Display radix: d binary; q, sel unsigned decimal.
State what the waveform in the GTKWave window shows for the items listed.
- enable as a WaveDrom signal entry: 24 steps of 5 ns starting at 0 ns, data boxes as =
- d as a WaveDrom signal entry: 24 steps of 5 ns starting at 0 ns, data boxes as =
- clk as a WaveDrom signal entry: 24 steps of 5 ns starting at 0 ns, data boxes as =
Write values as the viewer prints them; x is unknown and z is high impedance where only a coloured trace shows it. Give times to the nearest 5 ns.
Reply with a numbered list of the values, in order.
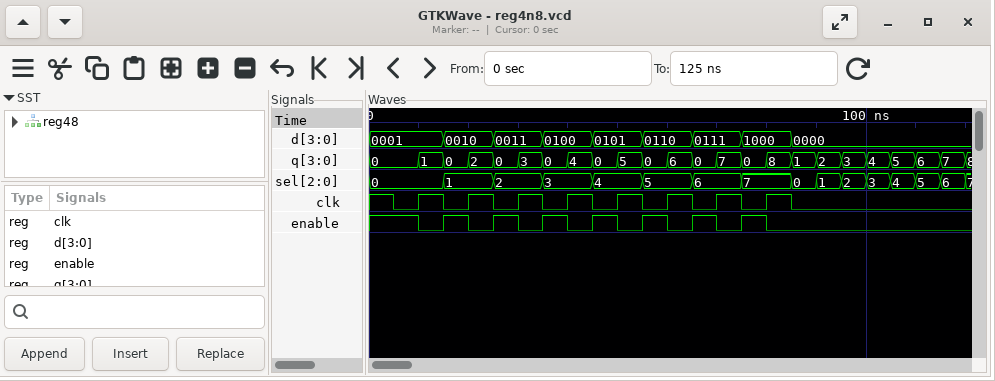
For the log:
1. {name: 'enable', wave: '1.010101010101010.......'}
2. {name: 'd', wave: '=..=.=.=.=.=.=.=.=......', data: '0001 0010 0011 0100 0101 0110 0111 1000 0000'}
3. {name: 'clk', wave: '101010101010101010......'}
